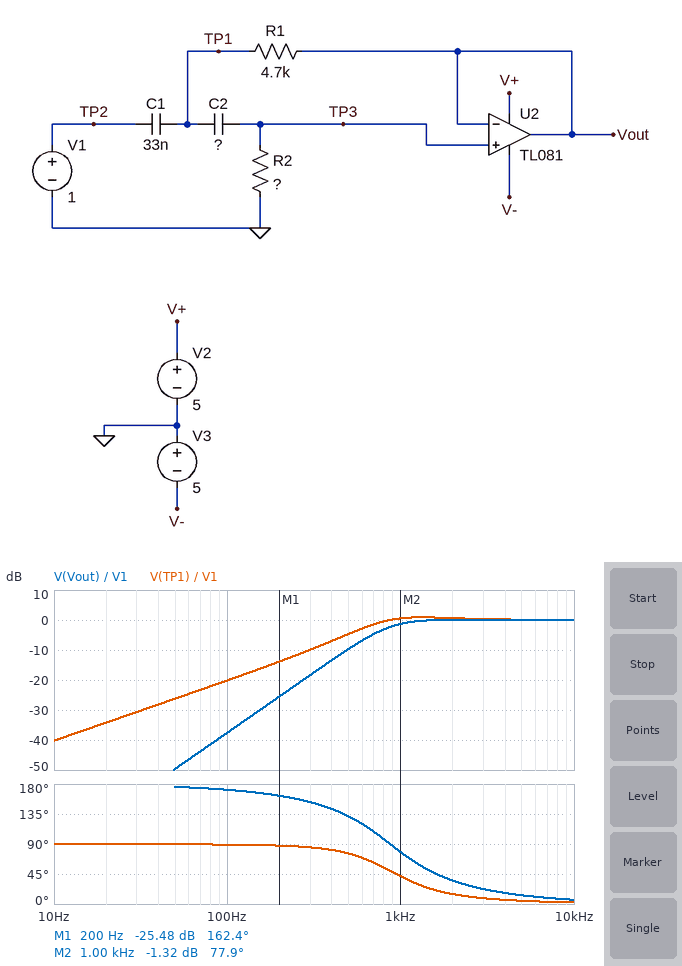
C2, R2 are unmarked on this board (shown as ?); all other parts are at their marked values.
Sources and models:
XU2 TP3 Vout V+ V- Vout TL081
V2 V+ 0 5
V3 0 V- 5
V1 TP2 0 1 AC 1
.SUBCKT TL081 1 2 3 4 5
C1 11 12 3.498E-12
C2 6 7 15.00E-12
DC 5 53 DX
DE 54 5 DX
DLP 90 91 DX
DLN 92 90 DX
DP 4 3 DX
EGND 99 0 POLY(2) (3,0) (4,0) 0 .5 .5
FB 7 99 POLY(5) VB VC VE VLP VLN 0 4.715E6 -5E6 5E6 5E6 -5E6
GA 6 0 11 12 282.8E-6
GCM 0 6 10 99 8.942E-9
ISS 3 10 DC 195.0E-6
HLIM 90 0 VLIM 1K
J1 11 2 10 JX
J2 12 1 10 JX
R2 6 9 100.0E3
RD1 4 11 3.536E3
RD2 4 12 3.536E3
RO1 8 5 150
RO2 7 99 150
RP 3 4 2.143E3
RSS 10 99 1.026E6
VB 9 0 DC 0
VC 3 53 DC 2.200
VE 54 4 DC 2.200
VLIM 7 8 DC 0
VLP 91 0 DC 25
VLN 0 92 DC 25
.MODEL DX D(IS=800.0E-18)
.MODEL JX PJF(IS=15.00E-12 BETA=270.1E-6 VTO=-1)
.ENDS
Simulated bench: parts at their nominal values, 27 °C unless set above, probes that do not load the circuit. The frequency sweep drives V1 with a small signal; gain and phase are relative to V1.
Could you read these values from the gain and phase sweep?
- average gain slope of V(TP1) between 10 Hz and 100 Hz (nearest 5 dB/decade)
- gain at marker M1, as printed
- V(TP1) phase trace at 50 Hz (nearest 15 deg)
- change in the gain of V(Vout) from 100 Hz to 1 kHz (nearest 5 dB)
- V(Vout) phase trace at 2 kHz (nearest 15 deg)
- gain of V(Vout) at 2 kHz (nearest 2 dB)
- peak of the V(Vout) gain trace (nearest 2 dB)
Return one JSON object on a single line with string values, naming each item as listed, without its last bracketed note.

{"average gain slope of V(TP1) between 10 Hz and 100 Hz": "20 dB/decade", "gain at marker M1, as printed": "-25.48 dB", "V(TP1) phase trace at 50 Hz": "90 deg", "change in the gain of V(Vout) from 100 Hz to 1 kHz": "35 dB", "V(Vout) phase trace at 2 kHz": "30 deg", "gain of V(Vout) at 2 kHz": "0 dB", "peak of the V(Vout) gain trace": "0 dB"}
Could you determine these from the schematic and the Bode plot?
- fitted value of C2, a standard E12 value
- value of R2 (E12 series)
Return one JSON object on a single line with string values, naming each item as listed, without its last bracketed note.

{"fitted value of C2, a standard E12 value": "18 nF", "value of R2": "12 kΩ"}
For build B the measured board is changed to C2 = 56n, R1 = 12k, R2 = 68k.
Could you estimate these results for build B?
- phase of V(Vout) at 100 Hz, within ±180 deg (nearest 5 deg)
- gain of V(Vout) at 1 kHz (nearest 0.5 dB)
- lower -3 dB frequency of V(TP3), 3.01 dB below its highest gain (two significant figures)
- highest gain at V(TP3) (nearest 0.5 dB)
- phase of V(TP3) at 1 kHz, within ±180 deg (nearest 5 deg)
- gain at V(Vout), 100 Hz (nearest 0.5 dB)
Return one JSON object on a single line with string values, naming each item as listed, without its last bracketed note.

{"phase of V(Vout) at 100 Hz, within ±180 deg": "120 deg", "gain of V(Vout) at 1 kHz": "0 dB", "lower -3 dB frequency of V(TP3), 3.01 dB below its highest gain": "110 Hz", "highest gain at V(TP3)": "2.0 dB", "phase of V(TP3) at 1 kHz, within ±180 deg": "5 deg", "gain at V(Vout), 100 Hz": "-2.5 dB"}
